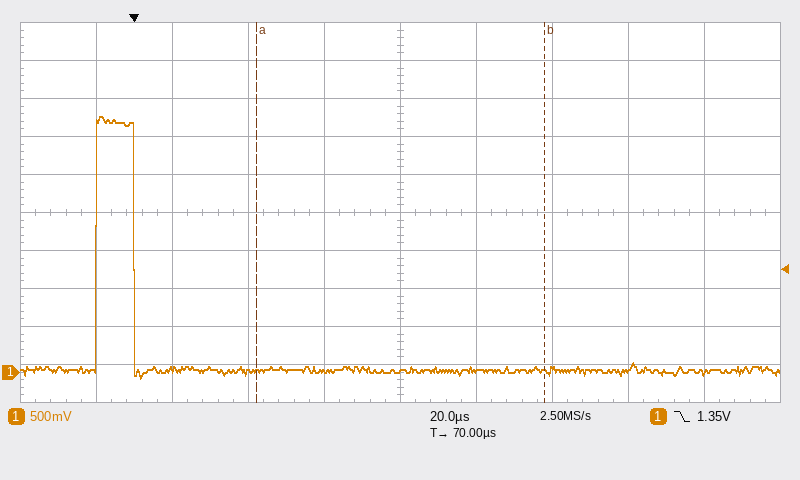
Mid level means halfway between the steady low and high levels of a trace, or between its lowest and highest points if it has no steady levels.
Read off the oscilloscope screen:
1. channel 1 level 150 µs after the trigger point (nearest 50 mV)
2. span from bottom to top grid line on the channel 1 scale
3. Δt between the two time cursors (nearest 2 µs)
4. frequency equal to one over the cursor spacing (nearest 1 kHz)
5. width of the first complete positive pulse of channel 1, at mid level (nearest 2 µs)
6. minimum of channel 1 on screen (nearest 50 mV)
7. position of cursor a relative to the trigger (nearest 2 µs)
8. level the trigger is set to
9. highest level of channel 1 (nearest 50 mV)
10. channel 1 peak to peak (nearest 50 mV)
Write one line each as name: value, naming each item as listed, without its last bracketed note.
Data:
channel 1 level 150 µs after the trigger point: 0 mV
span from bottom to top grid line on the channel 1 scale: 5 V
Δt between the two time cursors: 76 µs
frequency equal to one over the cursor spacing: 13 kHz
width of the first complete positive pulse of channel 1, at mid level: 10 µs
minimum of channel 1 on screen: -100 mV
position of cursor a relative to the trigger: +32 µs
level the trigger is set to: 1.35 V
highest level of channel 1: 3.35 V
channel 1 peak to peak: 3.45 V
